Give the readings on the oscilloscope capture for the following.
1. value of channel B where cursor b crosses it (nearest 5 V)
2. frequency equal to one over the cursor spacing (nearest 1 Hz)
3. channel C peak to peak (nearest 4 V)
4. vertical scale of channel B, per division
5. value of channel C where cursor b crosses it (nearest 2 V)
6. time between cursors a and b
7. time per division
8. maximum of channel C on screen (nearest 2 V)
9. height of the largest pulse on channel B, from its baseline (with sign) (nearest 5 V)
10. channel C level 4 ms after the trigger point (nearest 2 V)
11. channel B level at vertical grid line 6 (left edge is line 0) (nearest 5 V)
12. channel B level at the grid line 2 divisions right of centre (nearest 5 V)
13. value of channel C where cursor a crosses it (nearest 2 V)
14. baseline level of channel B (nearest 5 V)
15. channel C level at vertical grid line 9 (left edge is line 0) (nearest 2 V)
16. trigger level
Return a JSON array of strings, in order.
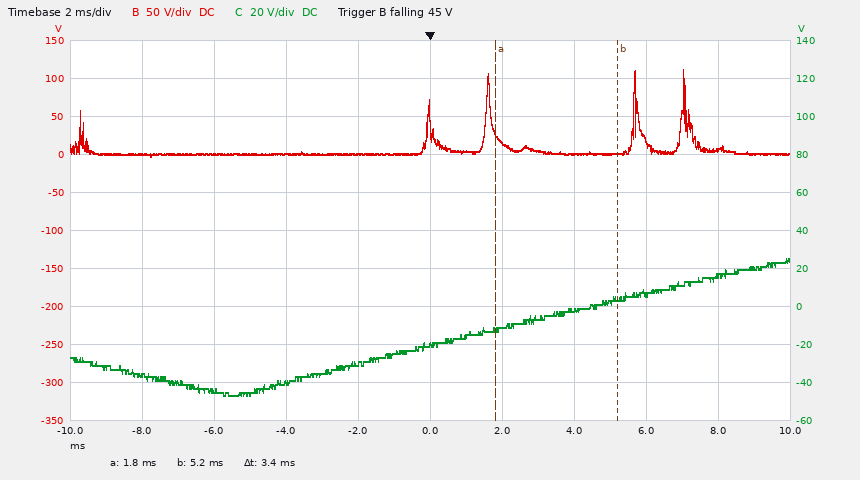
["0 V", "294 Hz", "72 V", "50 V", "4 V", "3.4 ms", "2 ms", "26 V", "+110 V", "-2 V", "15 V", "0 V", "-12 V", "0 V", "16 V", "45 V"]
